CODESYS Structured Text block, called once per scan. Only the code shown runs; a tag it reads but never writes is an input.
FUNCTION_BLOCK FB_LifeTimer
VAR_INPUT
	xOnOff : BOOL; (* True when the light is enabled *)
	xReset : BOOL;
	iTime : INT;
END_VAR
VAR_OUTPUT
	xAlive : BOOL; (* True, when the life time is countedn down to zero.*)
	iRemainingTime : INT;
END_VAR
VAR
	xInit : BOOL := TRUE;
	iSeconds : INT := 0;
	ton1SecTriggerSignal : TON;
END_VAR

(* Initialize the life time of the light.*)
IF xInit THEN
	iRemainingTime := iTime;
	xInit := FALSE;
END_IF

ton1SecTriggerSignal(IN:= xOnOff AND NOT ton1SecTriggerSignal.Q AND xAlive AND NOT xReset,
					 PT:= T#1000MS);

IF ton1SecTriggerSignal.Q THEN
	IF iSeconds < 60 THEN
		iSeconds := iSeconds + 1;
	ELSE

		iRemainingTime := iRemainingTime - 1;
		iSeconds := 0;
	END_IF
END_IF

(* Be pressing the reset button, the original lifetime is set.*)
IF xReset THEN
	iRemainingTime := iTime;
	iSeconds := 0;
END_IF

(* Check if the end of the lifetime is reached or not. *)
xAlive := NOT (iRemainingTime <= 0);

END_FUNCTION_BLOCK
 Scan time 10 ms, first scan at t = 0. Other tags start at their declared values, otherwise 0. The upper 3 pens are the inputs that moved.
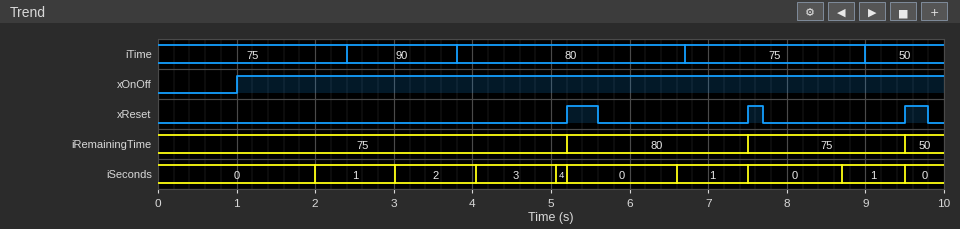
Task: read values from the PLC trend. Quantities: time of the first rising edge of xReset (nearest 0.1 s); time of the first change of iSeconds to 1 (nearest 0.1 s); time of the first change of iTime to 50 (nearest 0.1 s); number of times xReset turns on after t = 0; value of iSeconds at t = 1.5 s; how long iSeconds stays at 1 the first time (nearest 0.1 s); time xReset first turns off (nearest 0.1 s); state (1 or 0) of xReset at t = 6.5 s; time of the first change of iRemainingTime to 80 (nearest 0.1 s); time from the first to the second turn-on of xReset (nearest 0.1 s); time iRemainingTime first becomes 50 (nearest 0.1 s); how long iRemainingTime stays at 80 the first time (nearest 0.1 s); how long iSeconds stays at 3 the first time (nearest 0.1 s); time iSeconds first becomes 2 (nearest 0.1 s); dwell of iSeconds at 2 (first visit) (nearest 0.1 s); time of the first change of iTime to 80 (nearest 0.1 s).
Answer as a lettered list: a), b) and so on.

a) 5.2 s
b) 2.0 s
c) 9.0 s
d) 3
e) 0
f) 1.0 s
g) 5.6 s
h) 0
i) 5.2 s
j) 2.3 s
k) 9.5 s
l) 2.3 s
m) 1.0 s
n) 3.0 s
o) 1.0 s
p) 3.8 s
